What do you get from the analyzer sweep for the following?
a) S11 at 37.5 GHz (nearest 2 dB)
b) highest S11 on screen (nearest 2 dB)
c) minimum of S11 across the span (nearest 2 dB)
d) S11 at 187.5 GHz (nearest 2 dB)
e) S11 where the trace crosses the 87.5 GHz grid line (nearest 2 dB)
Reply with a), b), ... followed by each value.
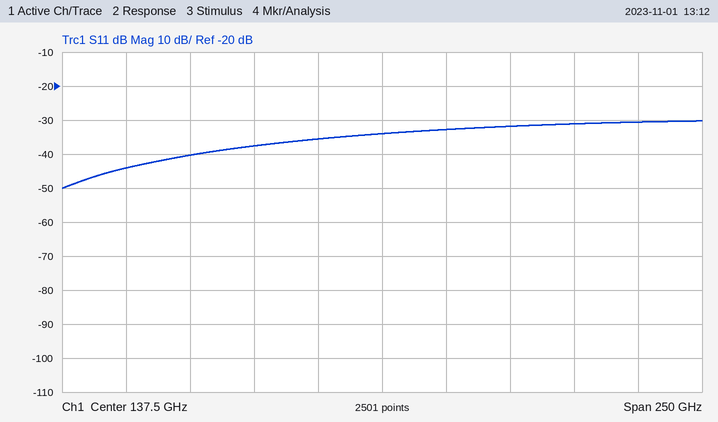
a) -44 dB
b) -30 dB
c) -50 dB
d) -32 dB
e) -38 dB
